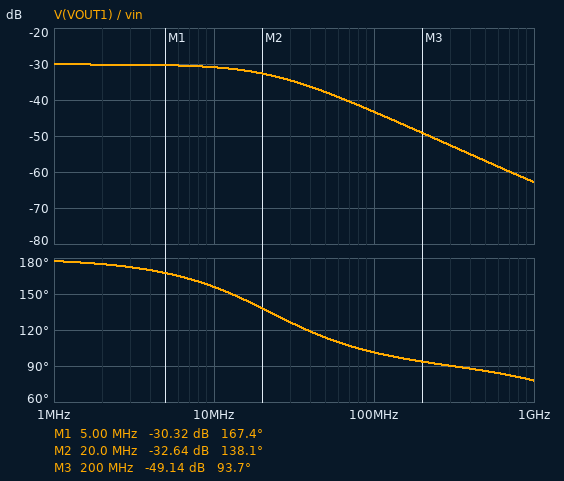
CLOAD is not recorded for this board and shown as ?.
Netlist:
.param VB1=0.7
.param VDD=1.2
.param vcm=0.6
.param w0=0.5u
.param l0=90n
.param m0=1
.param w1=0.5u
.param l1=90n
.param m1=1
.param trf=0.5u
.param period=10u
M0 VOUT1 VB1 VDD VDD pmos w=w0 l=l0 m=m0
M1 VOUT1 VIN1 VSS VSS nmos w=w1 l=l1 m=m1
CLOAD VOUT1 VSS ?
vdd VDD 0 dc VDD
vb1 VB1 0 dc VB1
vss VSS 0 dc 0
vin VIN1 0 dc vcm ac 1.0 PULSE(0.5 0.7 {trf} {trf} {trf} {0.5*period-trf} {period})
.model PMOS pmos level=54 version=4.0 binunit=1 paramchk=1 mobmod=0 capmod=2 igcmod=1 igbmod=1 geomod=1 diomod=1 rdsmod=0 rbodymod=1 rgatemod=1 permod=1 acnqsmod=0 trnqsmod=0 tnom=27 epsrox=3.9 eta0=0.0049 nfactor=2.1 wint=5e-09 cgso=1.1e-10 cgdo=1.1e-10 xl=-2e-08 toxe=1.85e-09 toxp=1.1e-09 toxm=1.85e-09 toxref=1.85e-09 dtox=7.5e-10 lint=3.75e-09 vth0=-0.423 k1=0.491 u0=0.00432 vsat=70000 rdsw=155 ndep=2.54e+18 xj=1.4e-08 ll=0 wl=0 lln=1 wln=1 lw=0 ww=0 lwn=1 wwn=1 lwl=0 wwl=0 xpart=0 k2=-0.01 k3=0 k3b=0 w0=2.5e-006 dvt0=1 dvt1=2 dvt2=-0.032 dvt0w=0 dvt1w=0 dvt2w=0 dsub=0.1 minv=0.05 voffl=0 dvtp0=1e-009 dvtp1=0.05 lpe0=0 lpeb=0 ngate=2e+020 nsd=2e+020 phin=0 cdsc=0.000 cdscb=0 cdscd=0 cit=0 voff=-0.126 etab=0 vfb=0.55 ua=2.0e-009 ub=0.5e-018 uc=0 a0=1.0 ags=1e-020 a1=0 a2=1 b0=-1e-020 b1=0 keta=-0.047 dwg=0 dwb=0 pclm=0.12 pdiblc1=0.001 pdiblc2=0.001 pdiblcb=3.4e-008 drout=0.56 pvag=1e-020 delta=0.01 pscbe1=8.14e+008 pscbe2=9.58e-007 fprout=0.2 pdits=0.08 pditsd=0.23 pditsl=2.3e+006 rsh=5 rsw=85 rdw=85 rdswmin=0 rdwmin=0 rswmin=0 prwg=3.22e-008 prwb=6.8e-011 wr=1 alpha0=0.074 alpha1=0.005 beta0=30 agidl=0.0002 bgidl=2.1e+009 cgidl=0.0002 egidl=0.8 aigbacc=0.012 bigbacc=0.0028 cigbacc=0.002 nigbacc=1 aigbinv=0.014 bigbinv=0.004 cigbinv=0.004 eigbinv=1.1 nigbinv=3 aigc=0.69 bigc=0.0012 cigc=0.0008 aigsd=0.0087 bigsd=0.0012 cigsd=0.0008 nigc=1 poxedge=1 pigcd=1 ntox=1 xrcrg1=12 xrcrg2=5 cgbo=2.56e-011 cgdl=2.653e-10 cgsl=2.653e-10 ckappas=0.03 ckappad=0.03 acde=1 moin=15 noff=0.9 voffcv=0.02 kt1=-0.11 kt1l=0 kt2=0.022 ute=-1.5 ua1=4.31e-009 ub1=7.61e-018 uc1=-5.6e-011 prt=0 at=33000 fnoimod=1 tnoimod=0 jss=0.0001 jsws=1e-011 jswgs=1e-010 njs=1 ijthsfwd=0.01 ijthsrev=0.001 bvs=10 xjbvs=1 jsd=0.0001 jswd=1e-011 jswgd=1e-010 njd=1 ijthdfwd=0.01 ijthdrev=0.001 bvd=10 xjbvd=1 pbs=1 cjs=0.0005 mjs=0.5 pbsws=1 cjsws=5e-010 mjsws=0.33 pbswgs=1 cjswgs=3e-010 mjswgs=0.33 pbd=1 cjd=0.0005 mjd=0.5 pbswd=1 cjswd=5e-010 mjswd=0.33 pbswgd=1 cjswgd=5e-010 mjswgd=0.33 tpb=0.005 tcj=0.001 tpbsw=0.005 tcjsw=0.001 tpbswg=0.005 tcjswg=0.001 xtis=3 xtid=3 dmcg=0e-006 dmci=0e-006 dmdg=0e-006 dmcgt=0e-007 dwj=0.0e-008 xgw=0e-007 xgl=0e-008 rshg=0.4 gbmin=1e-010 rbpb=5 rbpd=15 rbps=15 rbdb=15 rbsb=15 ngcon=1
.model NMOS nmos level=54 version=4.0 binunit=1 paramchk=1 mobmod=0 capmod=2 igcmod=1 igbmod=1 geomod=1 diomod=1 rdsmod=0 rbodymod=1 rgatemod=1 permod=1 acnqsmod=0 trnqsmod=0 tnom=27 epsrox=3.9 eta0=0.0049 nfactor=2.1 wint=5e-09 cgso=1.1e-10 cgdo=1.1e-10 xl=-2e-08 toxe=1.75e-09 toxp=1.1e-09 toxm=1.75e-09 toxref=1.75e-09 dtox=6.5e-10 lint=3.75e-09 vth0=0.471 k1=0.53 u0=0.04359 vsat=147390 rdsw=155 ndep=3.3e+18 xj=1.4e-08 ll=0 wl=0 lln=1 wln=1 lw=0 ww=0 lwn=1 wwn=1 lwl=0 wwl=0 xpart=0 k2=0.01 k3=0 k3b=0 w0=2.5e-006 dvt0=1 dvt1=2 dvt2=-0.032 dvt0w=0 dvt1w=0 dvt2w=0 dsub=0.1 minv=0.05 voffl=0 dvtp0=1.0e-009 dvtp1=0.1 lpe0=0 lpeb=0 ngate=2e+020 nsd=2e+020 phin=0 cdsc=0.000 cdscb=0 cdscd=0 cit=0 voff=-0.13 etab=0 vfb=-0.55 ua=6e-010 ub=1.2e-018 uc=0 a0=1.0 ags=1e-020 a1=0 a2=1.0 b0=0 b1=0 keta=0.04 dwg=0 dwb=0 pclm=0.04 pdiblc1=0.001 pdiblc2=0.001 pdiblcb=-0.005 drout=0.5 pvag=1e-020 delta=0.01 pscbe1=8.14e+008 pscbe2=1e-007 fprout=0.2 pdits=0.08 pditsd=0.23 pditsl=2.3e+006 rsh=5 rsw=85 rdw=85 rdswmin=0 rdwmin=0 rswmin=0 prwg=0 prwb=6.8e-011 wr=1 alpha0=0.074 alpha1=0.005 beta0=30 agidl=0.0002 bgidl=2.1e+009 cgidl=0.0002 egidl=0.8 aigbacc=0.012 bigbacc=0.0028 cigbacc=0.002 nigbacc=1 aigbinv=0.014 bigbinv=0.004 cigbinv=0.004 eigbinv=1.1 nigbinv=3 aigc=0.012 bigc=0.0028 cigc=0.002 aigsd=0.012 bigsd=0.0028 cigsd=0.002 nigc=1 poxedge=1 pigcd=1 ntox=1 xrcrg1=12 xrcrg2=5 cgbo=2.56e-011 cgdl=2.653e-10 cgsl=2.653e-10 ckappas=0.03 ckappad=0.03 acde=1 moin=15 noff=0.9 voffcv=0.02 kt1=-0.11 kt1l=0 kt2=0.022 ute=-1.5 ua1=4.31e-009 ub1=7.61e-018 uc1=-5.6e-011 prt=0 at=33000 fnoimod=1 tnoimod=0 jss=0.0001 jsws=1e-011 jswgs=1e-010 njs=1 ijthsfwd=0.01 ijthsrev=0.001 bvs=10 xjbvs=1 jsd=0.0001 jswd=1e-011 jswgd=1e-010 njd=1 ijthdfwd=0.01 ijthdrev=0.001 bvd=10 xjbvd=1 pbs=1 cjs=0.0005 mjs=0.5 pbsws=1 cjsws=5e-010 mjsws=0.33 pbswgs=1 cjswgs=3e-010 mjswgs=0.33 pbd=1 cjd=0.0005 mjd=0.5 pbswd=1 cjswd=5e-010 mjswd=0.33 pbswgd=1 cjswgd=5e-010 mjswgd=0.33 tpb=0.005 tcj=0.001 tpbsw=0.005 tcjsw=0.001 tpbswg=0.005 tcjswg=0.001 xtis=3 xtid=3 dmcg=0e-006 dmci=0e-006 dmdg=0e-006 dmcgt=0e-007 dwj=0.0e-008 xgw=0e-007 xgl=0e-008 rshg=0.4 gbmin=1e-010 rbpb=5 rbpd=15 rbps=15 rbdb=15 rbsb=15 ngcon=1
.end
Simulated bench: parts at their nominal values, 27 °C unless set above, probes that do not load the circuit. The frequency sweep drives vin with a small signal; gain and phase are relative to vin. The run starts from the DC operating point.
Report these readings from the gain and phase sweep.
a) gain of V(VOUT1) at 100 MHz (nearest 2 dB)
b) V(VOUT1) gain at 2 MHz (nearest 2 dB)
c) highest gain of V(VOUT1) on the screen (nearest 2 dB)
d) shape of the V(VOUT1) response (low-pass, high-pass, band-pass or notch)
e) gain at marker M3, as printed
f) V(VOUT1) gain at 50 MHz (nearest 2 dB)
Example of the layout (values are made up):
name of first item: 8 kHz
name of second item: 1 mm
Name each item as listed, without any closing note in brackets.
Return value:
gain of V(VOUT1) at 100 MHz: -44 dB
V(VOUT1) gain at 2 MHz: -30 dB
highest gain of V(VOUT1) on the screen: -30 dB
shape of the V(VOUT1) response: low-pass
gain at marker M3, as printed: -49.14 dB
V(VOUT1) gain at 50 MHz: -38 dB
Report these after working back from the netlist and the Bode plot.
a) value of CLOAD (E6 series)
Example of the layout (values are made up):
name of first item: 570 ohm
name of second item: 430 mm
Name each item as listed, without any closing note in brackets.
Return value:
value of CLOAD: 3.3 pF
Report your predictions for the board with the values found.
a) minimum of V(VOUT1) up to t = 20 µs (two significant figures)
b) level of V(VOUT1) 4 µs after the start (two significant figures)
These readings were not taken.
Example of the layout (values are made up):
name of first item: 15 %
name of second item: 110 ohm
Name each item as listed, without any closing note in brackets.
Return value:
minimum of V(VOUT1) up to t = 20 µs: 3.4 mV
level of V(VOUT1) 4 µs after the start: 3.4 mV
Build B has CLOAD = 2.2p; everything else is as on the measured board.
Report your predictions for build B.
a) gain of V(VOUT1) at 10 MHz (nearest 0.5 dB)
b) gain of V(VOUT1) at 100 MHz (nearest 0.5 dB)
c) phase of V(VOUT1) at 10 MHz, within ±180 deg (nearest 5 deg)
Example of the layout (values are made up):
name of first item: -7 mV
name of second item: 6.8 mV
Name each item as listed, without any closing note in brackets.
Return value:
gain of V(VOUT1) at 10 MHz: -30.5 dB
gain of V(VOUT1) at 100 MHz: -40.0 dB
phase of V(VOUT1) at 10 MHz, within ±180 deg: 165 deg
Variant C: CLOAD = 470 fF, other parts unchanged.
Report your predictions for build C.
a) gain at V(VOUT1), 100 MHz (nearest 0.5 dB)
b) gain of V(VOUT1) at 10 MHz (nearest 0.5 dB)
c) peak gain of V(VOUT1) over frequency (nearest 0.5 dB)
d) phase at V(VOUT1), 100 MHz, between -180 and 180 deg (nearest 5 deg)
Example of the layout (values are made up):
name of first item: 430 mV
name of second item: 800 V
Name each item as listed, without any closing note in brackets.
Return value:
gain at V(VOUT1), 100 MHz: -31.5 dB
gain of V(VOUT1) at 10 MHz: -30.0 dB
peak gain of V(VOUT1) over frequency: -30.0 dB
phase at V(VOUT1), 100 MHz, between -180 and 180 deg: 145 deg
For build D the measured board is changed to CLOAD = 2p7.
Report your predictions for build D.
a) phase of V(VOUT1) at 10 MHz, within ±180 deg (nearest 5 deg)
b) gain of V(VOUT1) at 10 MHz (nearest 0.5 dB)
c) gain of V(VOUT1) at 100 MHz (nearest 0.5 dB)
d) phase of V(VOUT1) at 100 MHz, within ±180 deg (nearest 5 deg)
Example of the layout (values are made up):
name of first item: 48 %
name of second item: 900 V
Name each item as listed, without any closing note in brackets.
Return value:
phase of V(VOUT1) at 10 MHz, within ±180 deg: 160 deg
gain of V(VOUT1) at 10 MHz: -30.5 dB
gain of V(VOUT1) at 100 MHz: -41.5 dB
phase of V(VOUT1) at 100 MHz, within ±180 deg: 105 deg
